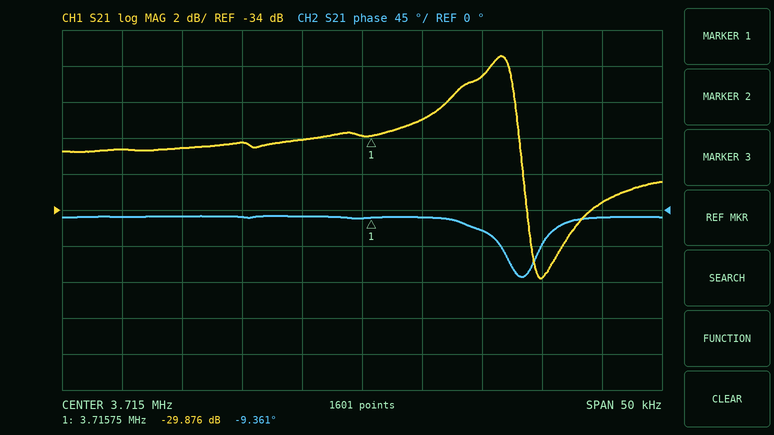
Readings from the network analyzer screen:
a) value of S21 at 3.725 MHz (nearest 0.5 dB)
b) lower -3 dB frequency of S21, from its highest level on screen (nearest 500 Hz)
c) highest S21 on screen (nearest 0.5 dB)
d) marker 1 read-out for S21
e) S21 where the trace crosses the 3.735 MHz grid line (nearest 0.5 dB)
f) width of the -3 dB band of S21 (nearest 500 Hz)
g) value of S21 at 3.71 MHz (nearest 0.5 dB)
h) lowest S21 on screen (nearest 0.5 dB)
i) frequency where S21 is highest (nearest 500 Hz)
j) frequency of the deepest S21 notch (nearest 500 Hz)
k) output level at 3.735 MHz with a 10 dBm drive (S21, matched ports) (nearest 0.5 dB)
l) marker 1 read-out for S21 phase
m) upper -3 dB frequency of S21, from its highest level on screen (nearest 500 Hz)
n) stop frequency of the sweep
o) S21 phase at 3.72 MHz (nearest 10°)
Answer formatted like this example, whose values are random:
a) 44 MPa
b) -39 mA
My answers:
a) -26.5 dB
b) 3.7215 MHz
c) -25.5 dB
d) -29.876 dB
e) -33.5 dB
f) 6.5 kHz
g) -30.0 dB
h) -38.0 dB
i) 3.7265 MHz
j) 3.7300 MHz
k) -23.5 dBm
l) -9.361°
m) 3.7280 MHz
n) 3.74 MHz
o) -10°
